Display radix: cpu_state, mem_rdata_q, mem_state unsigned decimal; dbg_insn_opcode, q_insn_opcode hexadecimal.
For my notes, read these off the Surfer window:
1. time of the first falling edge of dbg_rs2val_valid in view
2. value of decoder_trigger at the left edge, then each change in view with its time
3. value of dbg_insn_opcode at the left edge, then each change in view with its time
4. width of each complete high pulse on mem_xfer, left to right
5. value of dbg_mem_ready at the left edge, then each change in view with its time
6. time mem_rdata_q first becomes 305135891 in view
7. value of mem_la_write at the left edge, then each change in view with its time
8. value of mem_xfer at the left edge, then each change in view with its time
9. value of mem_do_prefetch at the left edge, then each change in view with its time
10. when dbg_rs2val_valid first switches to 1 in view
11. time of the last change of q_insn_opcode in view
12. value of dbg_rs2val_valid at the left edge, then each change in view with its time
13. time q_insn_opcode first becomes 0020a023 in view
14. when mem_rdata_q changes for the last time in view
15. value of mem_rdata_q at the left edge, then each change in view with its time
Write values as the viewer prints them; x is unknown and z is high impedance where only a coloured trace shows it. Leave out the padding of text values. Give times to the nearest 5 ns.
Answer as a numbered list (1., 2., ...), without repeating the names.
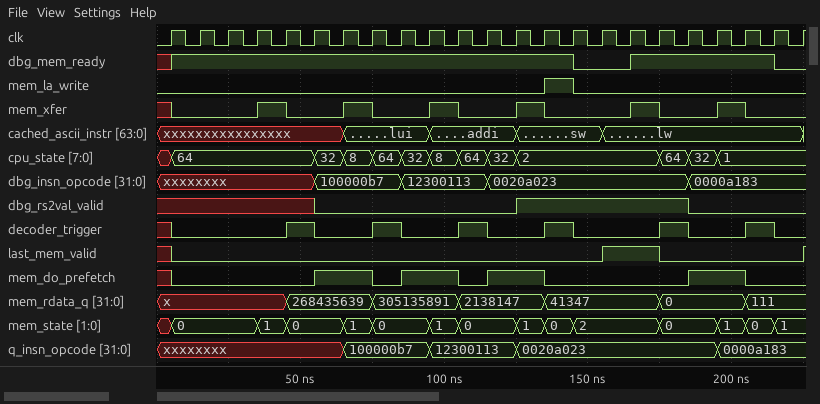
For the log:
1. 185 ns
2. x, 0 at 5 ns, 1 at 45 ns, 0 at 55 ns, 1 at 75 ns, 0 at 85 ns, 1 at 105 ns, 0 at 115 ns, 1 at 135 ns, 0 at 145 ns, 1 at 175 ns, 0 at 185 ns, 1 at 205 ns, 0 at 215 ns
3. xxxxxxxx, 100000b7 at 55 ns, 12300113 at 85 ns, 0020a023 at 115 ns, 0000a183 at 185 ns
4. 10 ns, 10 ns, 10 ns, 10 ns, 10 ns, 10 ns
5. x, 1 at 5 ns, 0 at 145 ns, 1 at 165 ns, 0 at 215 ns
6. 75 ns
7. 0, 1 at 135 ns, 0 at 145 ns
8. x, 0 at 5 ns, 1 at 35 ns, 0 at 45 ns, 1 at 65 ns, 0 at 75 ns, 1 at 95 ns, 0 at 105 ns, 1 at 125 ns, 0 at 135 ns, 1 at 165 ns, 0 at 175 ns, 1 at 195 ns, 0 at 205 ns
9. x, 0 at 5 ns, 1 at 55 ns, 0 at 75 ns, 1 at 85 ns, 0 at 105 ns, 1 at 115 ns, 0 at 135 ns, 1 at 185 ns, 0 at 205 ns
10. 125 ns
11. 195 ns
12. x, 0 at 55 ns, 1 at 125 ns, 0 at 185 ns
13. 125 ns
14. 205 ns
15. x, 268435639 at 45 ns, 305135891 at 75 ns, 2138147 at 105 ns, 41347 at 135 ns, 0 at 175 ns, 111 at 205 ns
